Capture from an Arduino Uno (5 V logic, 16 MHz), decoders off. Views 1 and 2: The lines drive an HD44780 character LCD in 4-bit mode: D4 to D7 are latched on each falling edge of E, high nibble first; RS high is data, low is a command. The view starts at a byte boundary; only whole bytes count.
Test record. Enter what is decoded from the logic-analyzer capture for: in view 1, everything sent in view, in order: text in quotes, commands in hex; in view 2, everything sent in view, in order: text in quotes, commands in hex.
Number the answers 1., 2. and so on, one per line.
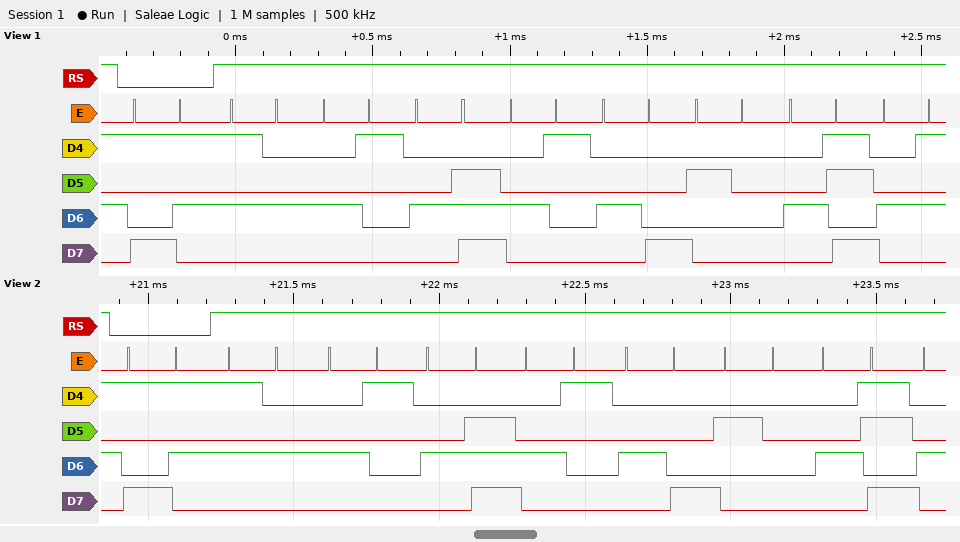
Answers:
1. 0x95 "TANAH KE"
2. 0x95 "TANAH K"
